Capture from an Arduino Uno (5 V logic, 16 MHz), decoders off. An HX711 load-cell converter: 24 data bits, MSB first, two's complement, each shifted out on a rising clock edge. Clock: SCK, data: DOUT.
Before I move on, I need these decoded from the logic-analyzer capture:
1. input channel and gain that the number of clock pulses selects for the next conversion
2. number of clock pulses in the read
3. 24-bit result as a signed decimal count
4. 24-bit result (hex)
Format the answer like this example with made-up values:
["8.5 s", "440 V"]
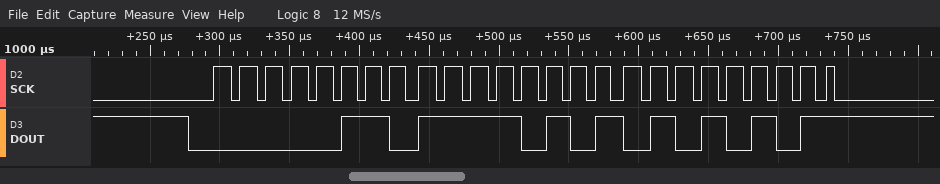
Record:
["channel A, gain 128", "25", "456021", "0x06F555"]
